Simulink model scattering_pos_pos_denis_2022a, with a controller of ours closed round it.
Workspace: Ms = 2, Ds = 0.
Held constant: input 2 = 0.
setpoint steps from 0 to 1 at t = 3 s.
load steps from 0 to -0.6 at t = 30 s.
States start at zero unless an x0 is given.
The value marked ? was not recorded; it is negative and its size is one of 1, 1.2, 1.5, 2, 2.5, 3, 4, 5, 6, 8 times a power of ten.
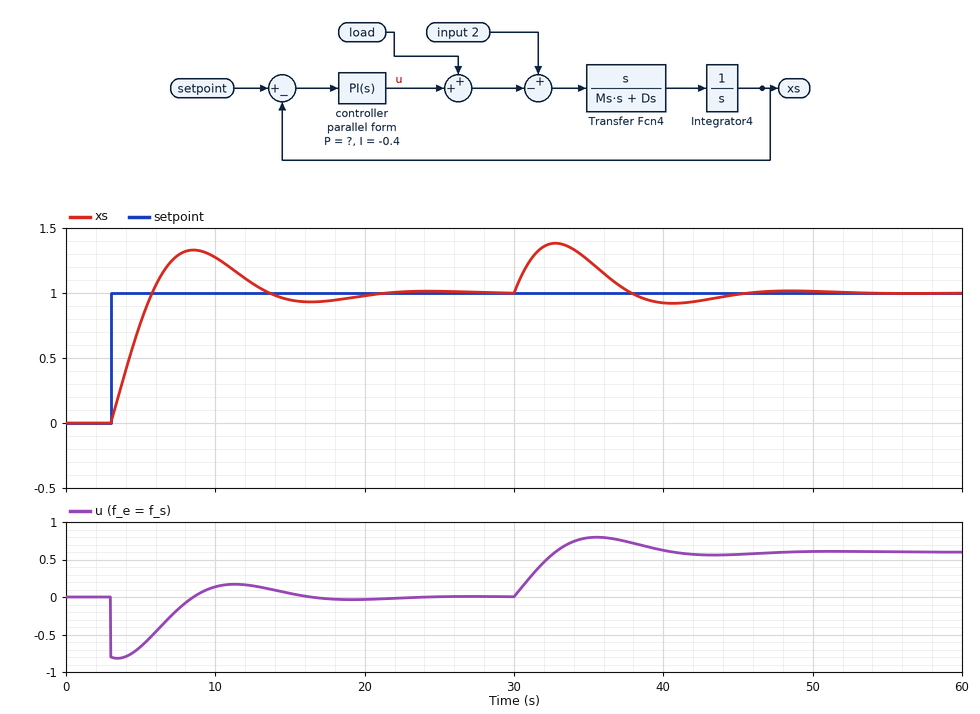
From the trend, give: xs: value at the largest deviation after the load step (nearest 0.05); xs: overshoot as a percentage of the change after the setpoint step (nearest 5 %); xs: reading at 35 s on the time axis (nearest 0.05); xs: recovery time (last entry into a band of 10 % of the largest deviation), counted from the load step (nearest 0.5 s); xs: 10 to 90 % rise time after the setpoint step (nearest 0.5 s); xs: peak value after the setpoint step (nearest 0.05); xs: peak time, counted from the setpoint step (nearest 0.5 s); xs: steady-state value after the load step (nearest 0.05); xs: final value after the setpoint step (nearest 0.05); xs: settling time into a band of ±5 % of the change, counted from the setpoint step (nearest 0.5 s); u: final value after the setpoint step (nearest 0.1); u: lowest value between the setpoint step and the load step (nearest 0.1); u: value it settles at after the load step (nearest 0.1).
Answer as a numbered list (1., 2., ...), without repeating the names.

1. 1.40
2. 35 %
3. 1.25
4. 13.5 s
5. 2.0 s
6. 1.35
7. 5.5 s
8. 1.00
9. 1.00
10. 15.5 s
11. 0.0
12. -0.8
13. 0.6
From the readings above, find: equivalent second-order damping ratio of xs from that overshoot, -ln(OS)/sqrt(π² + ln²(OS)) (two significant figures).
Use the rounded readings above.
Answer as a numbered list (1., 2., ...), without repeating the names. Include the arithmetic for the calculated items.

1. ln(0.35) = -1.050; 1.050 / sqrt(9.870 + 1.102) = 0.32
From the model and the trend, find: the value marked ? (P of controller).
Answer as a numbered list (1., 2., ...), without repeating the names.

1. -0.8
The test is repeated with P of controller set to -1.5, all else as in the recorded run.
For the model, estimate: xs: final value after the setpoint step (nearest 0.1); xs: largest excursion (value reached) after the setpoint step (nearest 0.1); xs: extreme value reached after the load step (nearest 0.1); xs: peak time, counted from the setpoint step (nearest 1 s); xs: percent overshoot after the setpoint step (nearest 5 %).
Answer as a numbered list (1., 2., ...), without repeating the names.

1. 1.0
2. 1.2
3. 1.3
4. 5 s
5. 15 %
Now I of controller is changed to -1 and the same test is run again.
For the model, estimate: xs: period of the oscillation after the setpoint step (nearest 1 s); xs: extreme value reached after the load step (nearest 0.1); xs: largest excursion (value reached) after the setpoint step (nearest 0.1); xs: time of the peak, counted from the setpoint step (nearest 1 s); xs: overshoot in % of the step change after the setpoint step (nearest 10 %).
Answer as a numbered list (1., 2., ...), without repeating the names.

1. 9 s
2. 1.3
3. 1.5
4. 4 s
5. 50 %
